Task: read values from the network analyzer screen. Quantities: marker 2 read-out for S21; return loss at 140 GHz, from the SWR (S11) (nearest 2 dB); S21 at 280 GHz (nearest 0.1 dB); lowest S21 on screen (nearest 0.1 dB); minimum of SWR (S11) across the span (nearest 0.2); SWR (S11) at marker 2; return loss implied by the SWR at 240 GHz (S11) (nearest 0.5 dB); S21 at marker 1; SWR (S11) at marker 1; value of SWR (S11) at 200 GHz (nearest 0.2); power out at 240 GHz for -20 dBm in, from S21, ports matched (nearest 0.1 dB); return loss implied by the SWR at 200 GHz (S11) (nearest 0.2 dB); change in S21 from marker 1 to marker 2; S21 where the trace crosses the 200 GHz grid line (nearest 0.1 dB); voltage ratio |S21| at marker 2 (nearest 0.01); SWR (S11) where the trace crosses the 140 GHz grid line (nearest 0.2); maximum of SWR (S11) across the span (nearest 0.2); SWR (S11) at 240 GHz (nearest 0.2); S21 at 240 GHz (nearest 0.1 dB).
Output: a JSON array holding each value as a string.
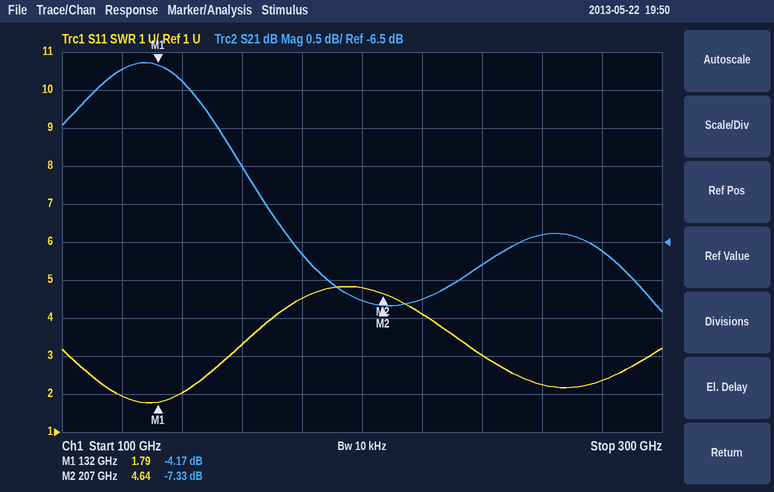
["-7.33 dB", "10 dB", "-6.6 dB", "-7.4 dB", "1.8", "4.64", "6.0 dB", "-4.17 dB", "1.79", "4.8", "-26.8 dBm", "3.6 dB", "-3.16 dB", "-7.3 dB", "0.43", "2.0", "4.8", "3.0", "-6.8 dB"]
